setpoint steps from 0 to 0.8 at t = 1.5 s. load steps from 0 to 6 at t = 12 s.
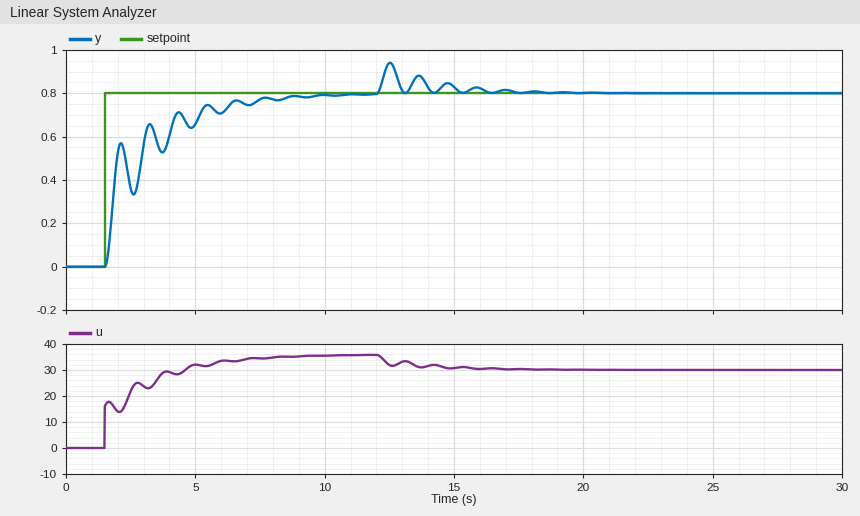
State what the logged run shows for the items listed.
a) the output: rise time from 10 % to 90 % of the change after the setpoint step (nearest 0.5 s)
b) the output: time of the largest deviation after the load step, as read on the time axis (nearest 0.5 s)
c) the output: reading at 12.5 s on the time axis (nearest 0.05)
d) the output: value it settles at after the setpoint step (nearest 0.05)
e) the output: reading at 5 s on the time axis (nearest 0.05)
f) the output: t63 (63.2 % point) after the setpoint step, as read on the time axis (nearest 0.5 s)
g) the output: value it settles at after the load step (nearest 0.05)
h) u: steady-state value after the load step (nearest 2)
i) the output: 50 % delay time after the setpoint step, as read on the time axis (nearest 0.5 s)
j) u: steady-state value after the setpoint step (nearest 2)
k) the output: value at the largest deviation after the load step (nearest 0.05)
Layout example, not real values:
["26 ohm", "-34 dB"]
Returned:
["3.5 s", "12.5 s", "0.95", "0.80", "0.65", "2.0 s", "0.80", "30", "2.0 s", "36", "0.95"]
